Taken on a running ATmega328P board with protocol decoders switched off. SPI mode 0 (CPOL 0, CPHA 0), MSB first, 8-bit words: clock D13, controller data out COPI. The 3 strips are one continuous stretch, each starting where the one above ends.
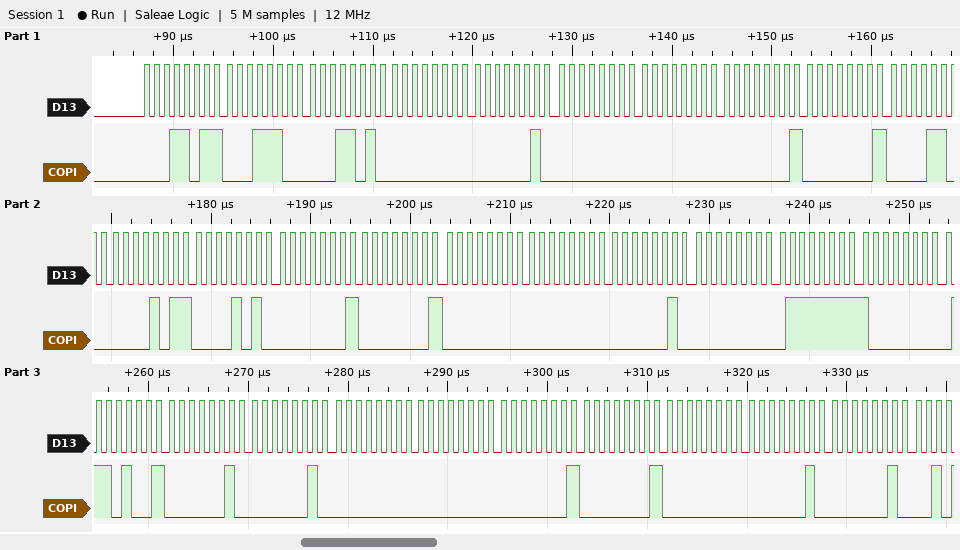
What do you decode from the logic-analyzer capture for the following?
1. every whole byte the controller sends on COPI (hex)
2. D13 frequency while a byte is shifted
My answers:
0x1B 0x1C 0x1A 0x00 0x02 0x00 0x00 0x01 0x01 0x0C 0x0B 0x0A 0x01 0x01 0x00 0x00 0x02 0x00 0x7F 0x80 0x69 0x02 0x02 0x00 0x00 0x01 0x01 0x00 0x02 0x02
1 MHz
